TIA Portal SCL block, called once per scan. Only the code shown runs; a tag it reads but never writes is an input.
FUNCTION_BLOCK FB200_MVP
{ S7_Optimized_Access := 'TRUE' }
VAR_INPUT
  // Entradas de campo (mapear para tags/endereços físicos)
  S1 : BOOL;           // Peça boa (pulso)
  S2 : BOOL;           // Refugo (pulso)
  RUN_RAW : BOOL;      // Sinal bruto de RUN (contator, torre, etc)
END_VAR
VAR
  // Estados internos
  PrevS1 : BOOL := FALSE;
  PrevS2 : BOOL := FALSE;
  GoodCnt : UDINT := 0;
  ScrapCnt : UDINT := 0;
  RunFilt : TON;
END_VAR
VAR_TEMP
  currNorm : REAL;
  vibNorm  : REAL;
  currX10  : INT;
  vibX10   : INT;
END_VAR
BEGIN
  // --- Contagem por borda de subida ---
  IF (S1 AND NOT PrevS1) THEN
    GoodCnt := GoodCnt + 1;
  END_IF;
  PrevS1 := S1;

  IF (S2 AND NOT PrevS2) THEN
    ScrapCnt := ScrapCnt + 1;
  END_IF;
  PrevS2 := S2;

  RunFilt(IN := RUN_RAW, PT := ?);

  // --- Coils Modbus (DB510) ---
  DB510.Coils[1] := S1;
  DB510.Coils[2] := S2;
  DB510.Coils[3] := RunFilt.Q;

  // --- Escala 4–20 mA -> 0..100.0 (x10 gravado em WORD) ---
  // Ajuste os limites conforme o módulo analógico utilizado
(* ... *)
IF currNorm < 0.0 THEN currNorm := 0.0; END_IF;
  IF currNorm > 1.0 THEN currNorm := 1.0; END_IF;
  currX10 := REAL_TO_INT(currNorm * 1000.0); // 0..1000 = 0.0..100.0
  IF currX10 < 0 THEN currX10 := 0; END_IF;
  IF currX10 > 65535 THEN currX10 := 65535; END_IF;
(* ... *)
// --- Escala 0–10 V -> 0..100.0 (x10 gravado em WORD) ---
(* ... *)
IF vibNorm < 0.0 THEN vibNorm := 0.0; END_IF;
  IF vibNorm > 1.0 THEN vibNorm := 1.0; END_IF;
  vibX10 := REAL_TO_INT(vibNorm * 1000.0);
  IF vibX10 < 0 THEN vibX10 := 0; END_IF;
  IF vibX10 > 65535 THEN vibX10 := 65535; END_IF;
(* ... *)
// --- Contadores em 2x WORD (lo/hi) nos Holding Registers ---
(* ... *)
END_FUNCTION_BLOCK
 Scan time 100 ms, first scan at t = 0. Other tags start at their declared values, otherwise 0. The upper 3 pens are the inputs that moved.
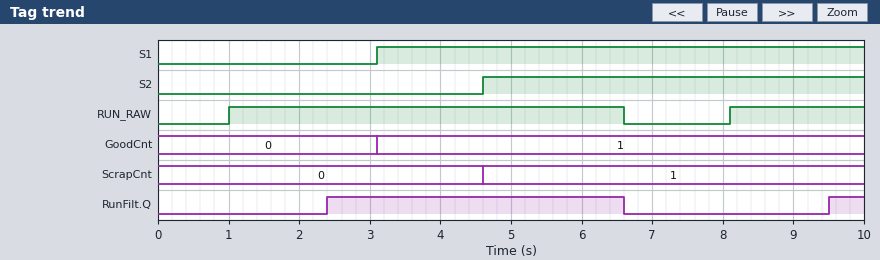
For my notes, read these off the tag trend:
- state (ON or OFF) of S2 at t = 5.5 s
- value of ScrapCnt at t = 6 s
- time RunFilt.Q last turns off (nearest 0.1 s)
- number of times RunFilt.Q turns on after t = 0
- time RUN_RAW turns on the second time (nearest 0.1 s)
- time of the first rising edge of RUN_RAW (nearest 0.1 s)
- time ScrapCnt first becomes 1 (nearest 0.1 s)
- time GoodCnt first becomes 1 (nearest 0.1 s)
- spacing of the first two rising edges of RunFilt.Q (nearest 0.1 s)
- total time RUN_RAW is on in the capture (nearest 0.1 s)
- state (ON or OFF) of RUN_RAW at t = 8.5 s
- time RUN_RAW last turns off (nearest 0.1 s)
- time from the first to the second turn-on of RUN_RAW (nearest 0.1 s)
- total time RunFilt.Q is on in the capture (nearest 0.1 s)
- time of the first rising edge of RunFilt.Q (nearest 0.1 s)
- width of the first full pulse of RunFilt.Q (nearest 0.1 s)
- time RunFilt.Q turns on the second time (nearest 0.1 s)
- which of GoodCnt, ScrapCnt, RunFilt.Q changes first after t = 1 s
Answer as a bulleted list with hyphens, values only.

- ON
- 1
- 6.6 s
- 2
- 8.1 s
- 1.0 s
- 4.6 s
- 3.1 s
- 7.1 s
- 7.5 s
- ON
- 6.6 s
- 7.1 s
- 4.7 s
- 2.4 s
- 4.2 s
- 9.5 s
- RunFilt.Q
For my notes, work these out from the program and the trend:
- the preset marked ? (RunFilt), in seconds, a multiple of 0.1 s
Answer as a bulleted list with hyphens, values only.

- 1.4 s
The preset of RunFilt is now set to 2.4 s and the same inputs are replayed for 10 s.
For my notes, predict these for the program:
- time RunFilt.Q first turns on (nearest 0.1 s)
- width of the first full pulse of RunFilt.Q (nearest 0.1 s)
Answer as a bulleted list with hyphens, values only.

- 3.4 s
- 3.2 s
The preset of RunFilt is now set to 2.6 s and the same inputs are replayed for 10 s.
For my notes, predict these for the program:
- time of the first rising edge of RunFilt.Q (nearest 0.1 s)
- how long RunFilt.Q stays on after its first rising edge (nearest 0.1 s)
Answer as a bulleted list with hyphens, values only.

- 3.6 s
- 3.0 s
